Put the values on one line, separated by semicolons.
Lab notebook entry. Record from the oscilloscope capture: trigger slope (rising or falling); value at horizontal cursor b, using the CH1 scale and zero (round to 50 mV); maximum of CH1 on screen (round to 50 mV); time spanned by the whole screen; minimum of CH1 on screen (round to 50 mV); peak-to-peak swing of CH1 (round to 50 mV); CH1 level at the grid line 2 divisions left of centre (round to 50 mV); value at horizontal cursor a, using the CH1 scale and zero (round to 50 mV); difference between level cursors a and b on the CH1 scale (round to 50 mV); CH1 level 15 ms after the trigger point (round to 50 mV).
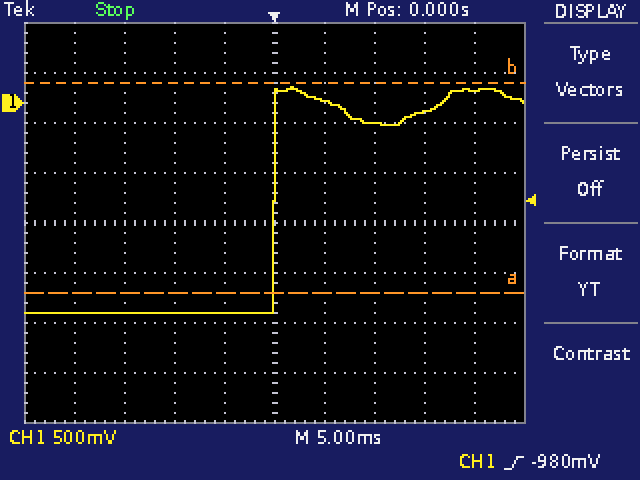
rising; 200 mV; 150 mV; 50 ms; -2.10 V; 2.25 V; -2.10 V; -1.90 V; 2.10 V; -100 mV
